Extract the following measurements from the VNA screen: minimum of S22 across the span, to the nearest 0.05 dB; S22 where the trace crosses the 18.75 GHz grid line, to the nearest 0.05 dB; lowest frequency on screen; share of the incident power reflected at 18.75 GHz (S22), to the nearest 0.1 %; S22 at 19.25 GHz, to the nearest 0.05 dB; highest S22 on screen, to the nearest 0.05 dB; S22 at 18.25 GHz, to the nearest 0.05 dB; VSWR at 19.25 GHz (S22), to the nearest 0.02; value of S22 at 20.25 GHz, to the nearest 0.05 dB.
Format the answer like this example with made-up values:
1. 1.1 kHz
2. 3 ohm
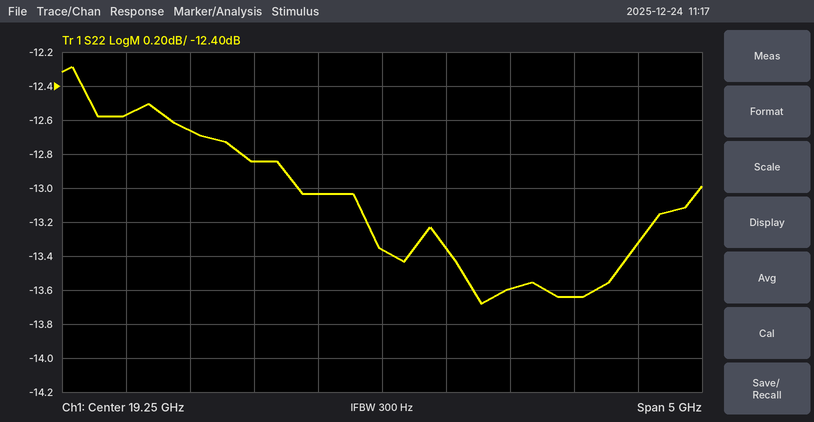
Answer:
1. -13.70 dB
2. -13.05 dB
3. 16.75 GHz
4. 5.0 %
5. -13.35 dB
6. -12.30 dB
7. -12.85 dB
8. 1.54
9. -13.60 dB
